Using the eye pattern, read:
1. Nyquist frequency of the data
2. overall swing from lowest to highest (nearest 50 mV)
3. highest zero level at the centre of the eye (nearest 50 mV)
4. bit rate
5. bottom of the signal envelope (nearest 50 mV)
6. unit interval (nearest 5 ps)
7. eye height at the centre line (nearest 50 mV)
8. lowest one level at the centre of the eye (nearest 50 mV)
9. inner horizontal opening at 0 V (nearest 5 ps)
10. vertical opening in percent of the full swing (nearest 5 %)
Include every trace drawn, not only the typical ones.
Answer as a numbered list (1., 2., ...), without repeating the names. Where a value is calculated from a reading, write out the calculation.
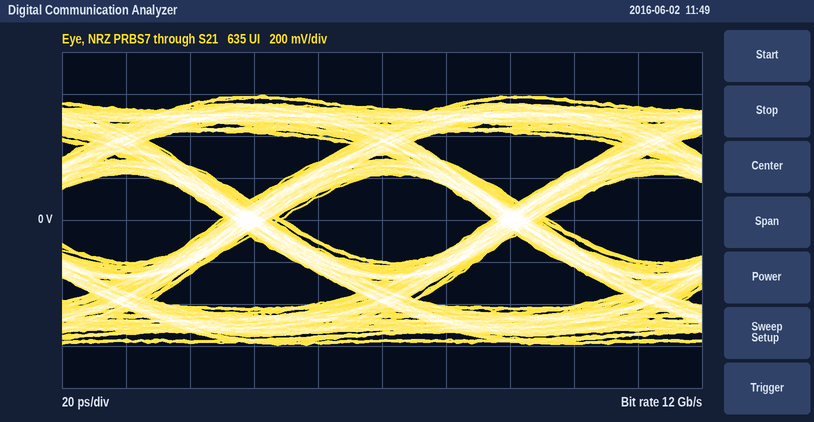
1. 6 GHz
2. 1.20 V
3. -200 mV
4. 12 Gb/s
5. -600 mV
6. 85 ps
7. 400 mV
8. 200 mV
9. 65 ps
10. 400 mV / 1.20 V ≈ 33.3 %, so 35 % to the nearest 5 %
